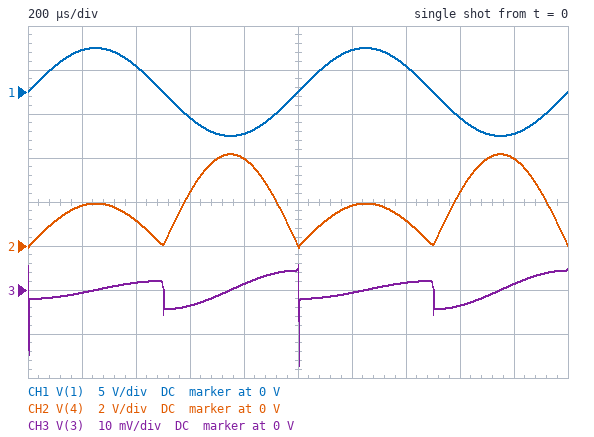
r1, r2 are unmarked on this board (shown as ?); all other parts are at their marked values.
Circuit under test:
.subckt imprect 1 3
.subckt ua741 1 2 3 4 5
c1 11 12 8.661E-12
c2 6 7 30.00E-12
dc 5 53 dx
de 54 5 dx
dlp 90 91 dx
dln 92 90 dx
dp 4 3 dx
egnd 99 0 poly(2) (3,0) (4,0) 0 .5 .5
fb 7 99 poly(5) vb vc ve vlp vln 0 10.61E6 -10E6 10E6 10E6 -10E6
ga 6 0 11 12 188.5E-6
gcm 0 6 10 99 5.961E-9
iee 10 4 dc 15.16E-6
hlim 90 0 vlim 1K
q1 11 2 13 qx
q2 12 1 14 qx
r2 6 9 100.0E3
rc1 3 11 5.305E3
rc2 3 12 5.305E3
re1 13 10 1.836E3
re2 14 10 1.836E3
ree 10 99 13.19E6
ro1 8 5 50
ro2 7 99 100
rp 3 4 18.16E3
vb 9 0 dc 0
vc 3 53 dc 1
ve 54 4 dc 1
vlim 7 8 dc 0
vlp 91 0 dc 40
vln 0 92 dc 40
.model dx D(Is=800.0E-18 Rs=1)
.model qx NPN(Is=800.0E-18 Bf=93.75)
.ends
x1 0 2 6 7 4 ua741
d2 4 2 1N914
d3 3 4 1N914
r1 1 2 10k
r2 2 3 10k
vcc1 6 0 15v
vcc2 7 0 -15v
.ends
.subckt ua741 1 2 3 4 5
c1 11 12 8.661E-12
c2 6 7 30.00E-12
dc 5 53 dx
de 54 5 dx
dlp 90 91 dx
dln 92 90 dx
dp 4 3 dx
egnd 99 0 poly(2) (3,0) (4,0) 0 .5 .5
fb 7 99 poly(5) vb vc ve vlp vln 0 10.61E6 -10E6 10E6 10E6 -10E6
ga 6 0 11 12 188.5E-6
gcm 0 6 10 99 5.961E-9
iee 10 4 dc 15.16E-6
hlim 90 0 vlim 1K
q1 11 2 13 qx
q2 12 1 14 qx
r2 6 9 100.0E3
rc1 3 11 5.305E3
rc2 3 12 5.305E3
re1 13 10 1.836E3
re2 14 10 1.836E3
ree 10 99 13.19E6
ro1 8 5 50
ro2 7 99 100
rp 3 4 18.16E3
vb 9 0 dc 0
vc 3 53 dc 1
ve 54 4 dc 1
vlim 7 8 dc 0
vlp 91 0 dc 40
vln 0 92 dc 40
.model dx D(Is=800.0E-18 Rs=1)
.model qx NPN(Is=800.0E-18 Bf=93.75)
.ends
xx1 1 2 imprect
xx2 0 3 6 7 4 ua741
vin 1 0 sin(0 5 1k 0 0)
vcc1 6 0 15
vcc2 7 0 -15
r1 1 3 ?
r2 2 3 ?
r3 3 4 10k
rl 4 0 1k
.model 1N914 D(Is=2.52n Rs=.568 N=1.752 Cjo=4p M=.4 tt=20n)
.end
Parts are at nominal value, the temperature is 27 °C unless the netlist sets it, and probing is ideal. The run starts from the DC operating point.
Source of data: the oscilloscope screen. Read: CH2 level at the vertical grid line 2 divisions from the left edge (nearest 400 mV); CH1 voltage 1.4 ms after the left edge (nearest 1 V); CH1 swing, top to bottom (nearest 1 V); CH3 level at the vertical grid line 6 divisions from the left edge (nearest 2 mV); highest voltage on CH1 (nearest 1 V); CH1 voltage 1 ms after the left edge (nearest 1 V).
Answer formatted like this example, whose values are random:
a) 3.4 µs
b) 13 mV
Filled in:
a) 1.2 V
b) 3 V
c) 10 V
d) 0 V
e) 5 V
f) 0 V
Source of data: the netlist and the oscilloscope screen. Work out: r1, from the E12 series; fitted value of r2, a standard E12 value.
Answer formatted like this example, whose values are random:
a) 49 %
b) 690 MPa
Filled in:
a) 12 kΩ
b) 8.2 kΩ
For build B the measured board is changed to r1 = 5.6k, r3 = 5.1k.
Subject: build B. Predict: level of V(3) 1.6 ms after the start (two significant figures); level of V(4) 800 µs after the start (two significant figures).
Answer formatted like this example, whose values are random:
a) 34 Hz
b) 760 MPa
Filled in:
a) -3.9 mV
b) 4.3 V
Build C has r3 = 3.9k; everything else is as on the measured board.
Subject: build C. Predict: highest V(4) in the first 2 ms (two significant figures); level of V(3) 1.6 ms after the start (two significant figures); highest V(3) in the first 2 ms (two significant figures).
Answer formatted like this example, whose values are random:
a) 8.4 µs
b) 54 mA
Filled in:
a) 1.6 V
b) -1.4 mV
c) 2.2 mV
